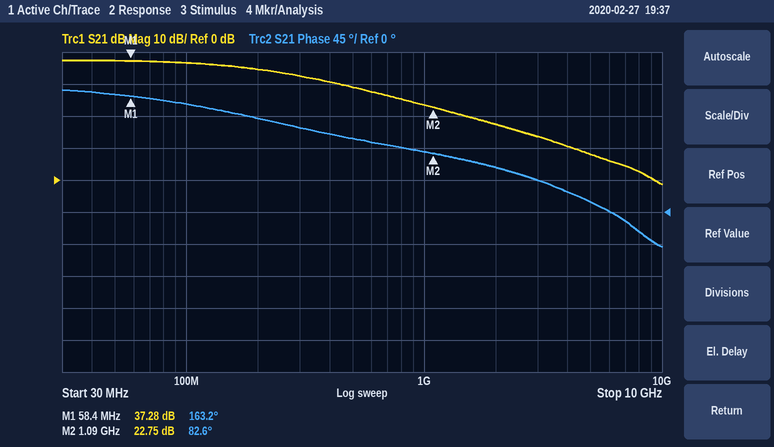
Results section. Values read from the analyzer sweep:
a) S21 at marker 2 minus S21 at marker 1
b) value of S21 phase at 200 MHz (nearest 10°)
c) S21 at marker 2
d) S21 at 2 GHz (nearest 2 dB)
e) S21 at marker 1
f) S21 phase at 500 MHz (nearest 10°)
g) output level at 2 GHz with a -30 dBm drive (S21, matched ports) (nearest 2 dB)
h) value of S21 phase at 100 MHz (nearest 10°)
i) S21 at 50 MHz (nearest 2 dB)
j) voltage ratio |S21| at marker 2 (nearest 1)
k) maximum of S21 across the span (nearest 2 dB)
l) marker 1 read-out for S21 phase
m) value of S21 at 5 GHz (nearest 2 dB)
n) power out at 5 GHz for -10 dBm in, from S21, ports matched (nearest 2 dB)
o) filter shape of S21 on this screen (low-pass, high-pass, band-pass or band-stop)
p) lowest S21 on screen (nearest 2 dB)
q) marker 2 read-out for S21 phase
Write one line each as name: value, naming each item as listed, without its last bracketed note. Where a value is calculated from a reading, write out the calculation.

S21 at marker 2 minus S21 at marker 1: 22.75 − (37.28) = -14.53 dB
value of S21 phase at 200 MHz: 130°
S21 at marker 2: 22.75 dB
S21 at 2 GHz: 18 dB
S21 at marker 1: 37.28 dB
S21 phase at 500 MHz: 100°
output level at 2 GHz with a -30 dBm drive (S21, matched ports): -30 dBm + (18 dB) = -12 dBm
value of S21 phase at 100 MHz: 150°
S21 at 50 MHz: 38 dB
voltage ratio |S21| at marker 2: 10^(22.75/20) ≈ 14
maximum of S21 across the span: 38 dB
marker 1 read-out for S21 phase: 163.2°
value of S21 at 5 GHz: 8 dB
power out at 5 GHz for -10 dBm in, from S21, ports matched: -10 dBm + (8 dB) = -2 dBm
filter shape of S21 on this screen: low-pass
lowest S21 on screen: -2 dB
marker 2 read-out for S21 phase: 82.6°
